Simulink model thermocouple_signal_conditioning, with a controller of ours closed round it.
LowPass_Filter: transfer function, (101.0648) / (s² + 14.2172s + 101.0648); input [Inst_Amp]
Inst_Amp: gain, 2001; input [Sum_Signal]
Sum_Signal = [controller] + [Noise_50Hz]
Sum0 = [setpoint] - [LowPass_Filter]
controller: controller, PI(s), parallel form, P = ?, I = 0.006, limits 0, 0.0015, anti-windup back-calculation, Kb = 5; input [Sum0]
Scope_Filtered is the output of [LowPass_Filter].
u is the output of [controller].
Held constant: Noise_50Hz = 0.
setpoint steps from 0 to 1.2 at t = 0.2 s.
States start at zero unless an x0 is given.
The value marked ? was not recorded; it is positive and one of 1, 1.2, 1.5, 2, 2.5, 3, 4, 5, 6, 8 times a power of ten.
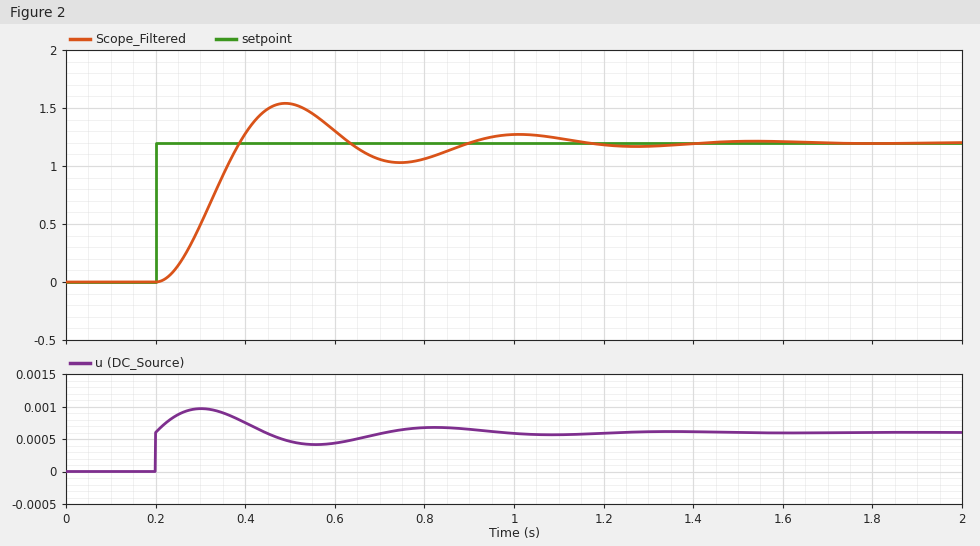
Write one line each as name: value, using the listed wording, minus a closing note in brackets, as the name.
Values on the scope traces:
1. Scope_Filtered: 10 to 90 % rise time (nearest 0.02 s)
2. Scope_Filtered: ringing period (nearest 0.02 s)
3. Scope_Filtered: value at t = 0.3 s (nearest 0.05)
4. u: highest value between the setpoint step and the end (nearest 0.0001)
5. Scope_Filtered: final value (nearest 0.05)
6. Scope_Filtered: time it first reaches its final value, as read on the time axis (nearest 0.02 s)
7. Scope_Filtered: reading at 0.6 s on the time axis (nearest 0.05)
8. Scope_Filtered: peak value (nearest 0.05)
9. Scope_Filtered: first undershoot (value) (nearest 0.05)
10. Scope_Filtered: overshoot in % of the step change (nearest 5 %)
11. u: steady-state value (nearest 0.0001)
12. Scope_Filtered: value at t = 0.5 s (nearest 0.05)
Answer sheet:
Scope_Filtered: 10 to 90 % rise time: 0.12 s
Scope_Filtered: ringing period: 0.52 s
Scope_Filtered: value at t = 0.3 s: 0.50
u: highest value between the setpoint step and the end: 0.0010
Scope_Filtered: final value: 1.20
Scope_Filtered: time it first reaches its final value, as read on the time axis: 0.38 s
Scope_Filtered: reading at 0.6 s on the time axis: 1.30
Scope_Filtered: peak value: 1.55
Scope_Filtered: first undershoot (value): 1.05
Scope_Filtered: overshoot in % of the step change: 30 %
u: steady-state value: 0.0006
Scope_Filtered: value at t = 0.5 s: 1.55
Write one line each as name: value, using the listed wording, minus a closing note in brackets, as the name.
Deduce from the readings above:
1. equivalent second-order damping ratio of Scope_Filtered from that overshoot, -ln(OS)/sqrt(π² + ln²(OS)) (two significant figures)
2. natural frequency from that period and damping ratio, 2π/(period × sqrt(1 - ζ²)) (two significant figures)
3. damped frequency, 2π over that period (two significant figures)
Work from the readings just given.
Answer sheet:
equivalent second-order damping ratio of Scope_Filtered from that overshoot, -ln(OS)/sqrt(π² + ln²(OS)): 0.36
natural frequency from that period and damping ratio, 2π/(period × sqrt(1 - ζ²)): 13 rad/s
damped frequency, 2π over that period: 12 rad/s
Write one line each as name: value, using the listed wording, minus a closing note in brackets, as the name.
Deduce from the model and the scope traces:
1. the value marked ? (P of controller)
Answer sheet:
the value marked ?: 0.0005
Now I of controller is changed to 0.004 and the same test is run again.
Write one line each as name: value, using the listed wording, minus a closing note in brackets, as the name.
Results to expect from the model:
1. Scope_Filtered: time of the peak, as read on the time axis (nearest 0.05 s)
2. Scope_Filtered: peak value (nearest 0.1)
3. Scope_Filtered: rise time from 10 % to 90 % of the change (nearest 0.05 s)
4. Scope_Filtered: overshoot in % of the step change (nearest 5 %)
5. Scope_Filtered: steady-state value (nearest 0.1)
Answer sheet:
Scope_Filtered: time of the peak, as read on the time axis: 0.50 s
Scope_Filtered: peak value: 1.3
Scope_Filtered: rise time from 10 % to 90 % of the change: 0.15 s
Scope_Filtered: overshoot in % of the step change: 10 %
Scope_Filtered: steady-state value: 1.2
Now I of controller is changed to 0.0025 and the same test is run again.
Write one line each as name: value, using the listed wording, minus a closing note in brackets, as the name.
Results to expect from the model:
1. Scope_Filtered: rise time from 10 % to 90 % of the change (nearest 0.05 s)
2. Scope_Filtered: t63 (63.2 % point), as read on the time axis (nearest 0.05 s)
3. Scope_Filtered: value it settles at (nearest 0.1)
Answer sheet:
Scope_Filtered: rise time from 10 % to 90 % of the change: 0.20 s
Scope_Filtered: t63 (63.2 % point), as read on the time axis: 0.35 s
Scope_Filtered: value it settles at: 1.2
